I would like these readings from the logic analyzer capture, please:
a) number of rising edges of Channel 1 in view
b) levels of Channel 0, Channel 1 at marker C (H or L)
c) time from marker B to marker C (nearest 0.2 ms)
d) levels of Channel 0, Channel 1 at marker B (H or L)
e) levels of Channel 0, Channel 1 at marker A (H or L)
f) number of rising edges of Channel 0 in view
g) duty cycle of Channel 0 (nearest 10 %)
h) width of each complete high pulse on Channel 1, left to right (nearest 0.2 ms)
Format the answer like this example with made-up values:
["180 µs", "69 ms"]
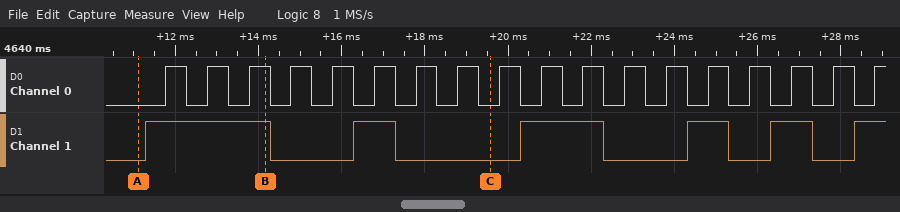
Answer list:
["6", "Channel 0=L, Channel 1=L", "5.4 ms", "Channel 0=H, Channel 1=H", "Channel 0=L, Channel 1=L", "18", "50 %", "3 ms, 1 ms, 2 ms, 1 ms, 1 ms"]
